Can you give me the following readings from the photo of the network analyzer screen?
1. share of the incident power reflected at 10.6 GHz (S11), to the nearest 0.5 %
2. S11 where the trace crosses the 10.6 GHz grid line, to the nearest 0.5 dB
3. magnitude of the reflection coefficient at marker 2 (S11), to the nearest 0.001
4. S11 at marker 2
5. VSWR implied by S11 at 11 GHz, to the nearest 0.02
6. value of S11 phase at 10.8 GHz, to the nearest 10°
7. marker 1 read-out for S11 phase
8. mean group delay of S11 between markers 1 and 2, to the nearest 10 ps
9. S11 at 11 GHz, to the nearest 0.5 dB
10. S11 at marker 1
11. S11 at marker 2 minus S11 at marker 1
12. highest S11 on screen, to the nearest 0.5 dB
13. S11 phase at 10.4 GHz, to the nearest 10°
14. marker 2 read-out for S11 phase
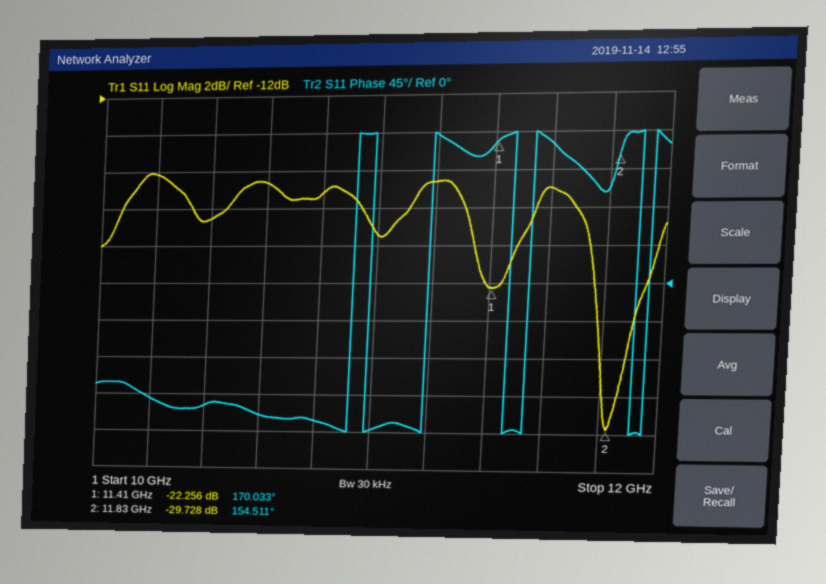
2.0 %
-16.5 dB
0.033
-29.728 dB
1.24
-170°
170.033°
100 ps
-19.5 dB
-22.256 dB
-7.472 dB
-16.0 dB
-150°
154.511°
